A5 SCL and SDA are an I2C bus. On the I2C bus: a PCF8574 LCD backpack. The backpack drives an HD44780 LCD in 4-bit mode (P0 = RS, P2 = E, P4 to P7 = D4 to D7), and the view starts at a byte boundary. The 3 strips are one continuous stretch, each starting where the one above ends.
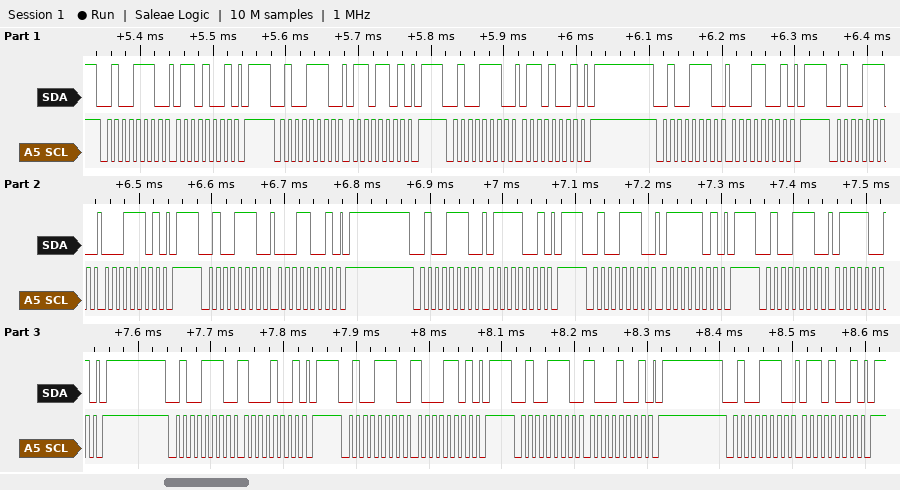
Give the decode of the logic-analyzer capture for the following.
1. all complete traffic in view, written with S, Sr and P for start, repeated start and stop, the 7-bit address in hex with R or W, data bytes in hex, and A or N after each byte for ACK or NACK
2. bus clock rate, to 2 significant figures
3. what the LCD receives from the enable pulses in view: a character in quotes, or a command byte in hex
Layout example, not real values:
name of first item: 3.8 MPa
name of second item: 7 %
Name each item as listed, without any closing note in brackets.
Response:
all complete traffic in view, written with S, Sr and P for start, repeated start and stop, the 7-bit address in hex with R or W, data bytes in hex, and A or N after each byte for ACK or NACK: S 27W A 69 A P S 27W A 6D A P S 27W A 69 A P S 27W A 19 A P S 27W A 1D A P S 27W A 19 A P S 27W A 79 A P S 27W A 7D A P S 27W A 79 A P S 27W A 89 A P S 27W A 8D A P S 27W A 89 A P S 27W A 69 A P
bus clock rate, to 2 significant figures: 100 kHz
what the LCD receives from the enable pulses in view: a character in quotes, or a command byte in hex: 'a' 'x'
